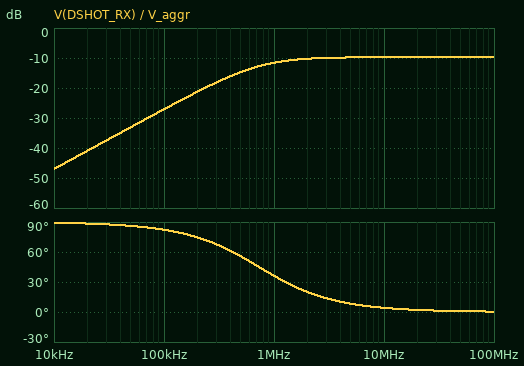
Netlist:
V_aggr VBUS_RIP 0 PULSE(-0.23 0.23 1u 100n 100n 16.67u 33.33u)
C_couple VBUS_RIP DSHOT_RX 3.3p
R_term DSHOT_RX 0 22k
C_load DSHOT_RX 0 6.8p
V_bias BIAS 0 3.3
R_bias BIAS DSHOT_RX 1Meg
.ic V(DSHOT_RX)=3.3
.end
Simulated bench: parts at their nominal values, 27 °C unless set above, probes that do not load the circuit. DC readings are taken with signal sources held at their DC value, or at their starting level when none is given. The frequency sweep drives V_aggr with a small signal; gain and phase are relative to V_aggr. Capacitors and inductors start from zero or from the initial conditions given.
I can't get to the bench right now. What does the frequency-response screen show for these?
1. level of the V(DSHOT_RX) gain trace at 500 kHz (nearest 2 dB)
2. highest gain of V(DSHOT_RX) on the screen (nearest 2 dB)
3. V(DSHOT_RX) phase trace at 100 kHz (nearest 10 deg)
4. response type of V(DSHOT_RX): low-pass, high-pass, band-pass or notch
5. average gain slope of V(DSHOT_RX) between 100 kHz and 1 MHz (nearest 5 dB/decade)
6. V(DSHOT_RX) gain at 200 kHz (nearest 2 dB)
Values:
-14 dB
-10 dB
80 deg
high-pass
15 dB/decade
-22 dB
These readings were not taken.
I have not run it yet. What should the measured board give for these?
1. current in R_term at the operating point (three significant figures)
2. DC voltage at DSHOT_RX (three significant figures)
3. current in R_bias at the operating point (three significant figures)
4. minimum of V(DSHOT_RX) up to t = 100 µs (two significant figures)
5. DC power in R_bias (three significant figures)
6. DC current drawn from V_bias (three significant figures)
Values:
3.23 µA
71.0 mV
3.23 µA
-50 mV
10.4 µW
3.23 µA
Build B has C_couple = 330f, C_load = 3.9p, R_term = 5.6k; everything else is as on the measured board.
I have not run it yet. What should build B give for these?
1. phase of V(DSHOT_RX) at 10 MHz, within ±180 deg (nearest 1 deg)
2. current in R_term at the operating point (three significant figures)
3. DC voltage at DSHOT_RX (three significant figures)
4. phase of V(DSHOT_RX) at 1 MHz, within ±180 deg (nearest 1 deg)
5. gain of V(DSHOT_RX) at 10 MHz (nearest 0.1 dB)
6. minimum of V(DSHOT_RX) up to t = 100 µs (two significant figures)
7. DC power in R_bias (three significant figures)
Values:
34 deg
3.28 µA
18.4 mV
82 deg
-23.8 dB
10 mV
10.8 µW
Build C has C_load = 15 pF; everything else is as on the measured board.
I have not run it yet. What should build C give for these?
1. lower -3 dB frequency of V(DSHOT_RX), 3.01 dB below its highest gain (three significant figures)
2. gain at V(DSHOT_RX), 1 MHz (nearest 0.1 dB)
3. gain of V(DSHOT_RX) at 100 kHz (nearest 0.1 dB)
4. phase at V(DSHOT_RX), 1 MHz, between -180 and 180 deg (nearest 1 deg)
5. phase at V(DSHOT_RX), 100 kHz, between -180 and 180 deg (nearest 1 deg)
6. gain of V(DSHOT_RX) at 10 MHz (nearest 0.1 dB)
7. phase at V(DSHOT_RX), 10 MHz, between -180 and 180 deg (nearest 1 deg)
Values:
404 kHz
-15.5 dB
-27.3 dB
22 deg
76 deg
-14.9 dB
2 deg
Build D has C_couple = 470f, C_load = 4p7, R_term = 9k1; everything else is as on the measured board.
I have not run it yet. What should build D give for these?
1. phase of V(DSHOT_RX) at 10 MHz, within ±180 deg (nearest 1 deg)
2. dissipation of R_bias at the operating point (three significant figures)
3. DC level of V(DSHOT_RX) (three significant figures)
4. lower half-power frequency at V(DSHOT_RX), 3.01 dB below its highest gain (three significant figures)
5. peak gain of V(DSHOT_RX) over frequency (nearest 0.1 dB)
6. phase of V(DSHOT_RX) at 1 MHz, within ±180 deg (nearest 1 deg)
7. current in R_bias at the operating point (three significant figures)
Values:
19 deg
10.7 µW
29.8 mV
3.41 MHz
-20.8 dB
74 deg
3.27 µA
